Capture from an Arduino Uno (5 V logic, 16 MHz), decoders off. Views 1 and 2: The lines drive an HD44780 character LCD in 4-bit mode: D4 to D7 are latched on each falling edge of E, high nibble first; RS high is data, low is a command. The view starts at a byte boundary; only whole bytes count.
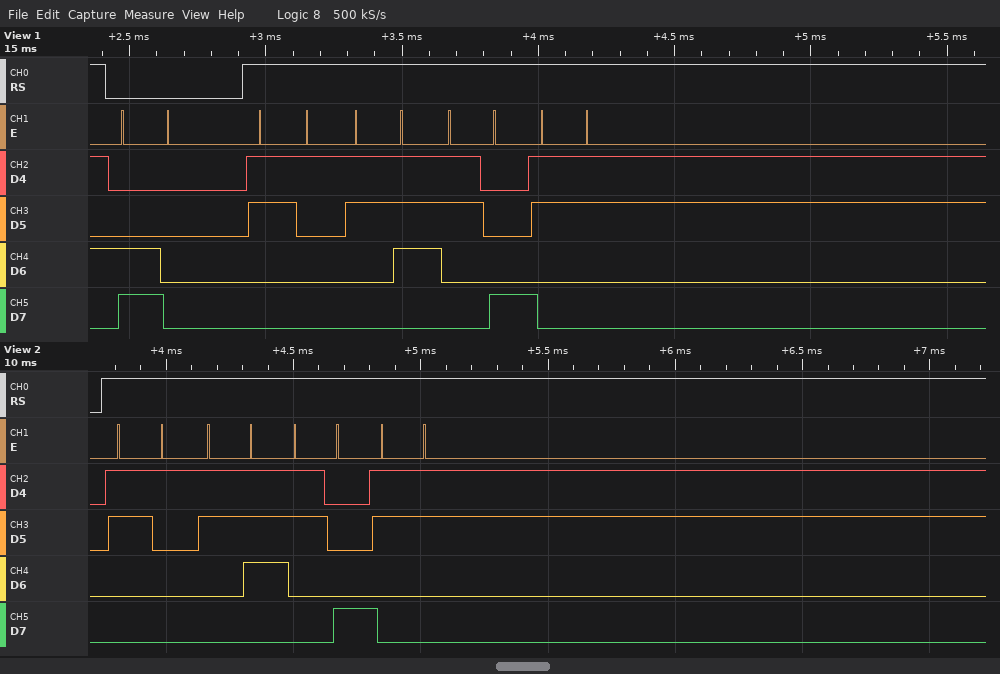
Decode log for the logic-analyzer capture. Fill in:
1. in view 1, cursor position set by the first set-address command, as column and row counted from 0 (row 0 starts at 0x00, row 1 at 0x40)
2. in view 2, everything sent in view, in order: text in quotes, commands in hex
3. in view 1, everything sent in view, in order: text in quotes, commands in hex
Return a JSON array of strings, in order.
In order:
["column 0, row 1", "\"1783\"", "0xC0 \"1783\""]
